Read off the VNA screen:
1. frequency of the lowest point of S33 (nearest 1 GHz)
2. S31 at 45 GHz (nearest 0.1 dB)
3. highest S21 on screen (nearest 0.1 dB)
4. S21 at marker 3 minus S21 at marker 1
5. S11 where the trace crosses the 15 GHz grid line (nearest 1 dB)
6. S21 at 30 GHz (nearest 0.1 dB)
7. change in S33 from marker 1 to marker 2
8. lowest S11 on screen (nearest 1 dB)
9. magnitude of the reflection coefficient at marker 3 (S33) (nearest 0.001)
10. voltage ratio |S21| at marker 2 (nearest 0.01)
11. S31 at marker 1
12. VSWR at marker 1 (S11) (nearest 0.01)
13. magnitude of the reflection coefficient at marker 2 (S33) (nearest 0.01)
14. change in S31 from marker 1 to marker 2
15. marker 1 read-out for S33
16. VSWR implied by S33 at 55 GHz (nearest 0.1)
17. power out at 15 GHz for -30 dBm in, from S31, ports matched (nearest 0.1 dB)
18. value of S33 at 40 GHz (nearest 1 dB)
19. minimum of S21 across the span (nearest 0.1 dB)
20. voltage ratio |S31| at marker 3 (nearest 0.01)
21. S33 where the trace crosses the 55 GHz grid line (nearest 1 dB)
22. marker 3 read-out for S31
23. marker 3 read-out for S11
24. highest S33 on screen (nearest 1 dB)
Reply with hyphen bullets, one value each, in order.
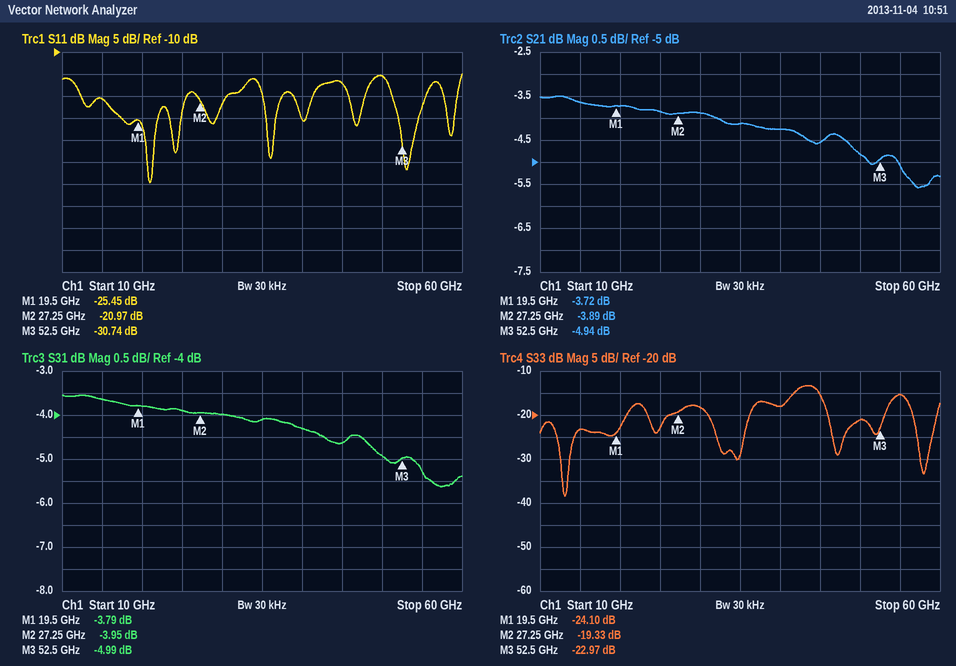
- 13 GHz
- -4.6 dB
- -3.5 dB
- -1.22 dB
- -21 dB
- -3.9 dB
- 4.77 dB
- -40 dB
- 0.071
- 0.64
- -3.79 dB
- 1.11
- 0.11
- -0.16 dB
- -24.10 dB
- 1.4
- -33.6 dBm
- -18 dB
- -5.6 dB
- 0.56
- -15 dB
- -4.99 dB
- -30.74 dB
- -13 dB
